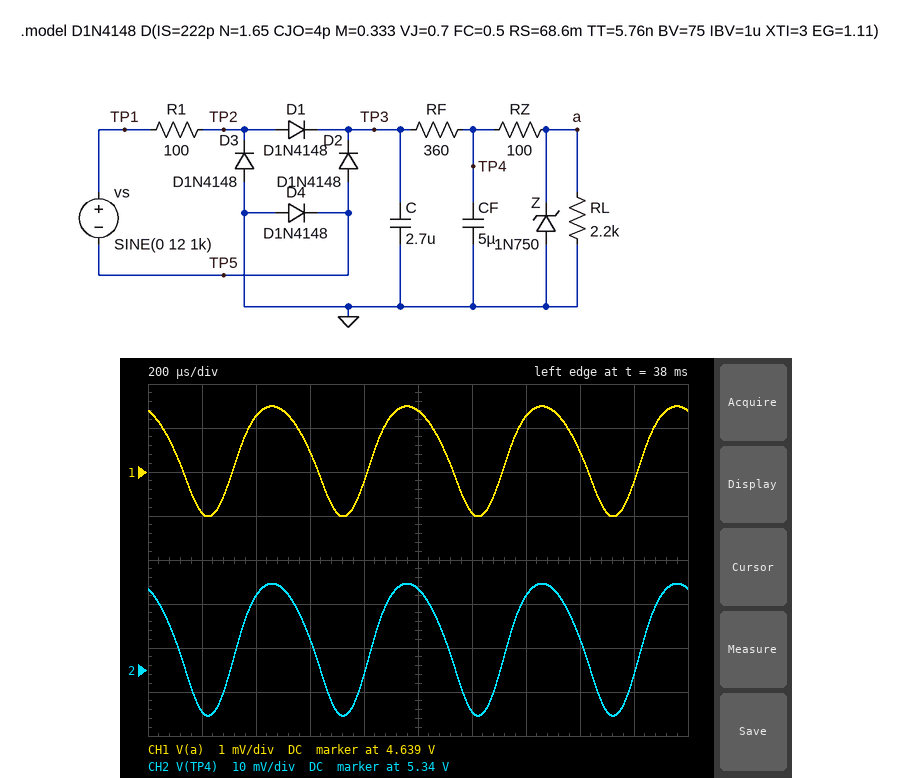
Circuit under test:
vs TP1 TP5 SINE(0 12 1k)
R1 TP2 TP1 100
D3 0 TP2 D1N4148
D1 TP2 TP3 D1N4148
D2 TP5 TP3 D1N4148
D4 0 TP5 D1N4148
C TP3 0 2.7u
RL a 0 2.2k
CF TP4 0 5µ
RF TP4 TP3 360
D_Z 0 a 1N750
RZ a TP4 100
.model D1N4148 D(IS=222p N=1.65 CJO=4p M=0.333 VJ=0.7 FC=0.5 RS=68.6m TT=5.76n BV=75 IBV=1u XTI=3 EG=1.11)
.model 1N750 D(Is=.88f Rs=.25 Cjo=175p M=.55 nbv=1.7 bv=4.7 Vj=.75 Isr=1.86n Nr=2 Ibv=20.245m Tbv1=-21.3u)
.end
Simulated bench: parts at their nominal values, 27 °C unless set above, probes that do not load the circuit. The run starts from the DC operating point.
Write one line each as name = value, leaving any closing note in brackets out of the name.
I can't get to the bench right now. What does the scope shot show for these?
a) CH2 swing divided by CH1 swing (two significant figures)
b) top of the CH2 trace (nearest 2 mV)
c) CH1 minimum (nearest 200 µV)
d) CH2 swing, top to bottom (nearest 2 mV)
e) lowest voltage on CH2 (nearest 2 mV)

CH2 swing divided by CH1 swing = 12
top of the CH2 trace = 5.360 V
CH1 minimum = 4.6380 V
CH2 swing, top to bottom = 30 mV
lowest voltage on CH2 = 5.330 V
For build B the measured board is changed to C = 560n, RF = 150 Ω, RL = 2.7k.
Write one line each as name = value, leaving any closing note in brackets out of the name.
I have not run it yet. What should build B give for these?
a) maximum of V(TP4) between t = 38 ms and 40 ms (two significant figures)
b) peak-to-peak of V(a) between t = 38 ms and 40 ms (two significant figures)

maximum of V(TP4) between t = 38 ms and 40 ms = 5.7 V
peak-to-peak of V(a) between t = 38 ms and 40 ms = 17 mV
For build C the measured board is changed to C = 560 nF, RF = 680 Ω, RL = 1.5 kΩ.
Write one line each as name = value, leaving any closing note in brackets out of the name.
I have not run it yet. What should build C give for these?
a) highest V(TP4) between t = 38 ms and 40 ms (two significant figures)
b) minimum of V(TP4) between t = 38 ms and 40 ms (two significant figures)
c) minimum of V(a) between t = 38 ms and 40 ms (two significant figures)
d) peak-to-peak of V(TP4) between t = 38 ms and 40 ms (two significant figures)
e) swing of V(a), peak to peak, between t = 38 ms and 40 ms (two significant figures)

highest V(TP4) between t = 38 ms and 40 ms = 5.1 V
minimum of V(TP4) between t = 38 ms and 40 ms = 5.0 V
minimum of V(a) between t = 38 ms and 40 ms = 4.6 V
peak-to-peak of V(TP4) between t = 38 ms and 40 ms = 51 mV
swing of V(a), peak to peak, between t = 38 ms and 40 ms = 11 mV
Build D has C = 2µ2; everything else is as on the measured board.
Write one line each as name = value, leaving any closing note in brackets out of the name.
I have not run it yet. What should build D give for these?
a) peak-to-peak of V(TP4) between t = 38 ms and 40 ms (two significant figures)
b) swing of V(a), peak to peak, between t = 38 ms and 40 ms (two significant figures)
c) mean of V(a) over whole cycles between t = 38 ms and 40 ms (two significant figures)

peak-to-peak of V(TP4) between t = 38 ms and 40 ms = 37 mV
swing of V(a), peak to peak, between t = 38 ms and 40 ms = 3.1 mV
mean of V(a) over whole cycles between t = 38 ms and 40 ms = 4.6 V
